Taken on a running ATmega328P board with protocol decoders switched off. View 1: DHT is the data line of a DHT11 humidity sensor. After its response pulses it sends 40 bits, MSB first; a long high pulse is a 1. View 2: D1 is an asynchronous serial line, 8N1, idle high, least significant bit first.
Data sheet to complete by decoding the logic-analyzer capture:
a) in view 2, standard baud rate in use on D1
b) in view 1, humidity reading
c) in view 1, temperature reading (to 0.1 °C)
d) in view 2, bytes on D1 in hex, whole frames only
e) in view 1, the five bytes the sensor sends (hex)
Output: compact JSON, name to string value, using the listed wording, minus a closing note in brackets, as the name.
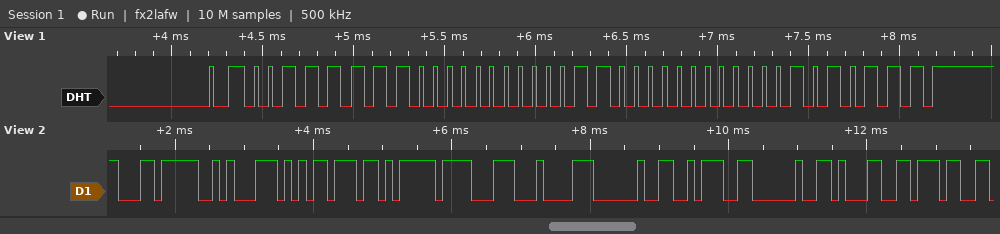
{"in view 2, standard baud rate in use on D1": "9600 baud", "in view 1, humidity reading": "63 %", "in view 1, temperature reading": "24.0 °C", "in view 2, bytes on D1 in hex, whole frames only": "0xEC 0x8A 0xB5 0xEB 0x8F 0x84 0x20 0x3A 0x20 0x31 0x37", "in view 1, the five bytes the sensor sends": "3F 00 18 00 57"}
